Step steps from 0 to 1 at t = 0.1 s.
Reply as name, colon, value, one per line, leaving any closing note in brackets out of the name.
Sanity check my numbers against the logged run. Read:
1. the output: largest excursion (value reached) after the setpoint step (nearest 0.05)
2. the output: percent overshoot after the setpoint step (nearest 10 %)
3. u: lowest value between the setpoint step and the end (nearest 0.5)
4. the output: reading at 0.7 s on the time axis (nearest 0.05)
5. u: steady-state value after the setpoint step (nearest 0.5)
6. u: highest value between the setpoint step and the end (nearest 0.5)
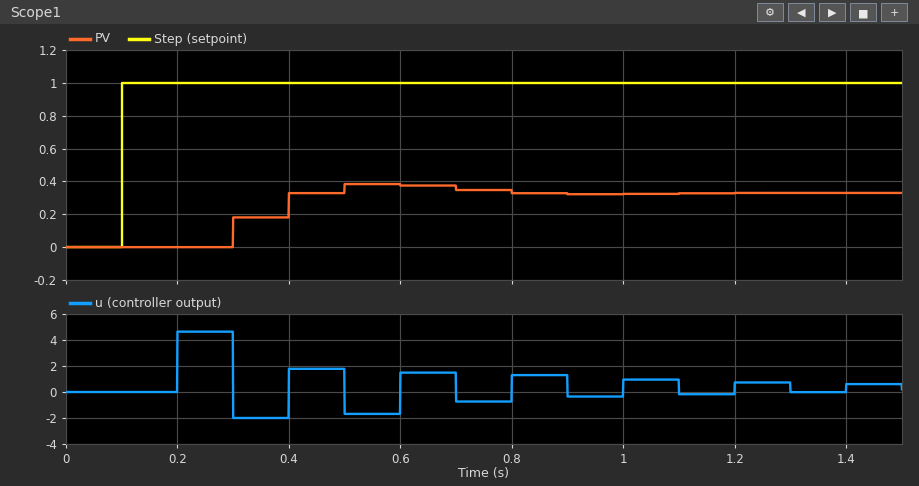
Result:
the output: largest excursion (value reached) after the setpoint step: 0.40
the output: percent overshoot after the setpoint step: 20 %
u: lowest value between the setpoint step and the end: -2.0
the output: reading at 0.7 s on the time axis: 0.35
u: steady-state value after the setpoint step: 0.5
u: highest value between the setpoint step and the end: 4.5
